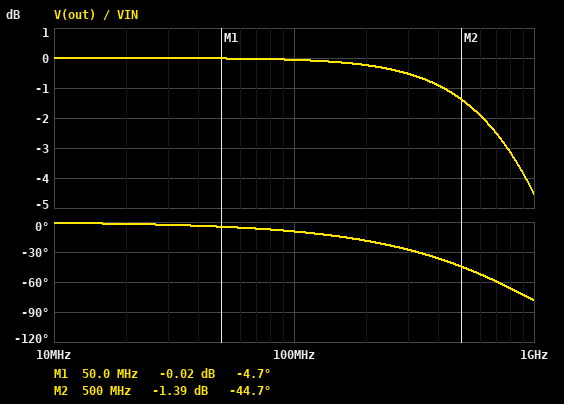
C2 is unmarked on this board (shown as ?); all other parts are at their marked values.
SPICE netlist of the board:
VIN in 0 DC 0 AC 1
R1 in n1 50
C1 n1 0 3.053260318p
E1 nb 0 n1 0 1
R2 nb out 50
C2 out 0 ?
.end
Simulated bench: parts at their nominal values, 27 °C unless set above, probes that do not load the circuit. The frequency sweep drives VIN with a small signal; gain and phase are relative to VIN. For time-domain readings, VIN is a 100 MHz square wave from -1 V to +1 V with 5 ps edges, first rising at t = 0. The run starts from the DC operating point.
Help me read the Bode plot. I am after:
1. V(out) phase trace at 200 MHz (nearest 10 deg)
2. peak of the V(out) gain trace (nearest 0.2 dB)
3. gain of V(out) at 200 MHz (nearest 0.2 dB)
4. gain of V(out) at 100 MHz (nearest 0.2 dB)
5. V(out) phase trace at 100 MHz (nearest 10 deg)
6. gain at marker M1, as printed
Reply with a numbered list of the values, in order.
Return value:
1. -20 deg
2. 0 dB
3. -0.2 dB
4. 0 dB
5. -10 deg
6. -0.02 dB
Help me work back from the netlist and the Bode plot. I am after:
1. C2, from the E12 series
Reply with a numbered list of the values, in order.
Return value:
1. 2.2 pF
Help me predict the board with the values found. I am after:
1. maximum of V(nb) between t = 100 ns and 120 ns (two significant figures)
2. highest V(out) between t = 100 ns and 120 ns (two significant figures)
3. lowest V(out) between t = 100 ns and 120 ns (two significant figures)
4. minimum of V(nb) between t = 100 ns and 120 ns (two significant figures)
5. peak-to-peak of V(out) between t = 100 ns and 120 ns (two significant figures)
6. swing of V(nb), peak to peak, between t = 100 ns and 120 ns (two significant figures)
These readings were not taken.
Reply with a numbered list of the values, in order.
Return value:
1. 1.0 V
2. 1.0 V
3. -1.0 V
4. -1.0 V
5. 2.0 V
6. 2.0 V
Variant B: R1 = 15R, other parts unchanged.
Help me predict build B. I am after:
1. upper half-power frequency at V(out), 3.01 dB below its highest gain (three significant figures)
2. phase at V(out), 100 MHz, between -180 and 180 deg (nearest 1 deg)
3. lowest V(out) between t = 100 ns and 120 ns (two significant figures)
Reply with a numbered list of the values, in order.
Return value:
1. 1.27 GHz
2. -6 deg
3. -1.0 V
